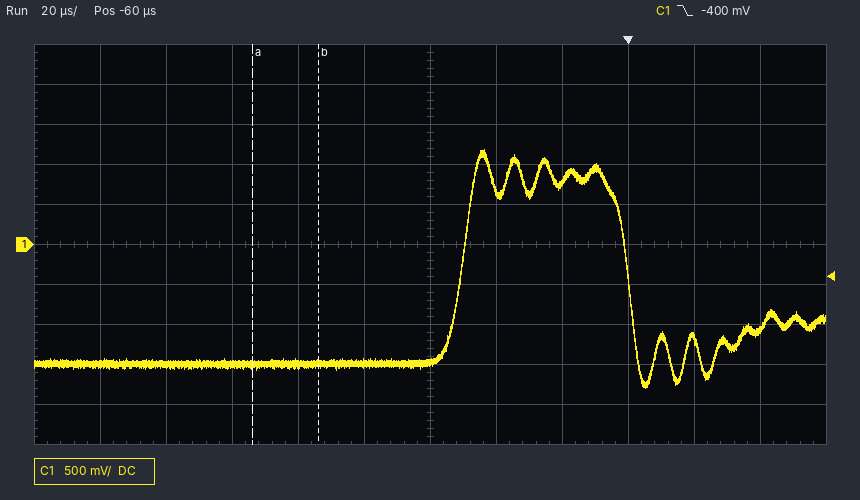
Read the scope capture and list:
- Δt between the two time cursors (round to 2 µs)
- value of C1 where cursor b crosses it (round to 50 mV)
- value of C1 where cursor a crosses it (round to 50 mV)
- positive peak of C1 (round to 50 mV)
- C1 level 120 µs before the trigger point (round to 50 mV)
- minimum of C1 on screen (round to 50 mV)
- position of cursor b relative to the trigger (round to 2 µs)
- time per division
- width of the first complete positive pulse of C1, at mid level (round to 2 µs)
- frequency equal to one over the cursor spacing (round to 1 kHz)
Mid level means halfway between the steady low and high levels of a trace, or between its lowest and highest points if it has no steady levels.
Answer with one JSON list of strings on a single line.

["20 µs", "-1.50 V", "-1.50 V", "1.20 V", "-1.50 V", "-1.80 V", "-94 µs", "20 µs", "50 µs", "50 kHz"]
